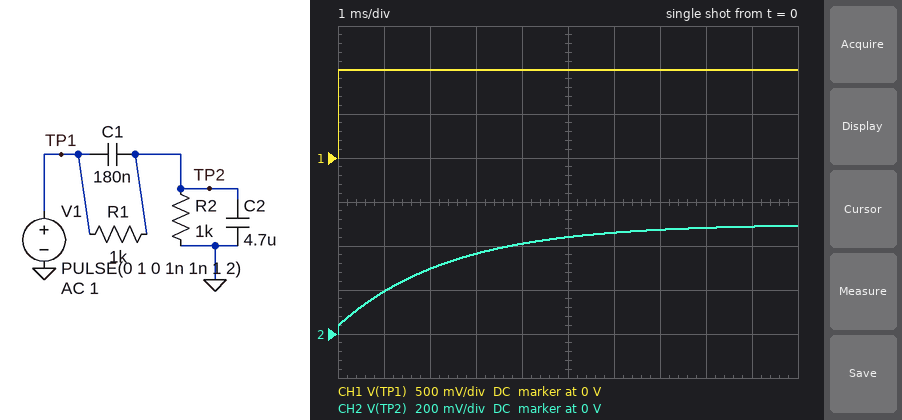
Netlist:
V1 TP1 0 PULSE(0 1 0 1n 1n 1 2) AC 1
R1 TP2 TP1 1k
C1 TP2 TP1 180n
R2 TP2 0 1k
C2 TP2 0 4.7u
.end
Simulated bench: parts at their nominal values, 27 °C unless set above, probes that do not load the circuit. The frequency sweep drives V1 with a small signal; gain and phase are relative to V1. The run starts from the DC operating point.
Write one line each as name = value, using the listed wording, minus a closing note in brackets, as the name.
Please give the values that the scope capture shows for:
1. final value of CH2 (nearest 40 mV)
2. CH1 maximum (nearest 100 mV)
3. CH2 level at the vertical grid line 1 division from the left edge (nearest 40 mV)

final value of CH2 = 480 mV
CH1 maximum = 1.0 V
CH2 level at the vertical grid line 1 division from the left edge = 200 mV
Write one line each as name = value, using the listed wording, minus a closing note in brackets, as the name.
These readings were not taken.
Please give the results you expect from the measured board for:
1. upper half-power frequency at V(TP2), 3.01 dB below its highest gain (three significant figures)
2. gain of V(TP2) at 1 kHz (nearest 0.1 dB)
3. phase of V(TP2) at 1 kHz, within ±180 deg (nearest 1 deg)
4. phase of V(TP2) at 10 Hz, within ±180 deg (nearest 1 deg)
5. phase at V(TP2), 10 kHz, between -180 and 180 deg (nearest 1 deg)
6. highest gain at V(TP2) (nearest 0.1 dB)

upper half-power frequency at V(TP2), 3.01 dB below its highest gain = 65.6 Hz
gain of V(TP2) at 1 kHz = -26.2 dB
phase of V(TP2) at 1 kHz, within ±180 deg = -38 deg
phase of V(TP2) at 10 Hz, within ±180 deg = -8 deg
phase at V(TP2), 10 kHz, between -180 and 180 deg = -5 deg
highest gain at V(TP2) = -6.0 dB
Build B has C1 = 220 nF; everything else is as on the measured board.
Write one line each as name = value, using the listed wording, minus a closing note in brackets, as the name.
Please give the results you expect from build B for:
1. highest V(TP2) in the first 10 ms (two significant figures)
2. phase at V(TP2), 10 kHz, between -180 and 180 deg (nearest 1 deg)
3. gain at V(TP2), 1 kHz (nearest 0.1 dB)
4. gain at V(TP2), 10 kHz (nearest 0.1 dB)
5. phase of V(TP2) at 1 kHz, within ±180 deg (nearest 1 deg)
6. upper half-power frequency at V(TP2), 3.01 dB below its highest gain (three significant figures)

highest V(TP2) in the first 10 ms = 490 mV
phase at V(TP2), 10 kHz, between -180 and 180 deg = -4 deg
gain at V(TP2), 1 kHz = -25.2 dB
gain at V(TP2), 10 kHz = -27.0 dB
phase of V(TP2) at 1 kHz, within ±180 deg = -32 deg
upper half-power frequency at V(TP2), 3.01 dB below its highest gain = 65.2 Hz
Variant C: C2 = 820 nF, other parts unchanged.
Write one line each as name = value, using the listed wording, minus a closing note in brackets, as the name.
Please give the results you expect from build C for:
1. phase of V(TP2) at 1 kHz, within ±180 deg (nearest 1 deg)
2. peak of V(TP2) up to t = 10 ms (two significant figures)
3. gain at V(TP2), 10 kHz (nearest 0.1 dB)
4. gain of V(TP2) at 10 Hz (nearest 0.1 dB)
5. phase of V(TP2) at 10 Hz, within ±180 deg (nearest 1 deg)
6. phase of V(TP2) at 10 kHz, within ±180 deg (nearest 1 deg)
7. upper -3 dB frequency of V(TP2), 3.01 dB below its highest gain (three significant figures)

phase of V(TP2) at 1 kHz, within ±180 deg = -24 deg
peak of V(TP2) up to t = 10 ms = 500 mV
gain at V(TP2), 10 kHz = -14.9 dB
gain of V(TP2) at 10 Hz = -6.0 dB
phase of V(TP2) at 10 Hz, within ±180 deg = -1 deg
phase of V(TP2) at 10 kHz, within ±180 deg = -3 deg
upper -3 dB frequency of V(TP2), 3.01 dB below its highest gain = 370 Hz
